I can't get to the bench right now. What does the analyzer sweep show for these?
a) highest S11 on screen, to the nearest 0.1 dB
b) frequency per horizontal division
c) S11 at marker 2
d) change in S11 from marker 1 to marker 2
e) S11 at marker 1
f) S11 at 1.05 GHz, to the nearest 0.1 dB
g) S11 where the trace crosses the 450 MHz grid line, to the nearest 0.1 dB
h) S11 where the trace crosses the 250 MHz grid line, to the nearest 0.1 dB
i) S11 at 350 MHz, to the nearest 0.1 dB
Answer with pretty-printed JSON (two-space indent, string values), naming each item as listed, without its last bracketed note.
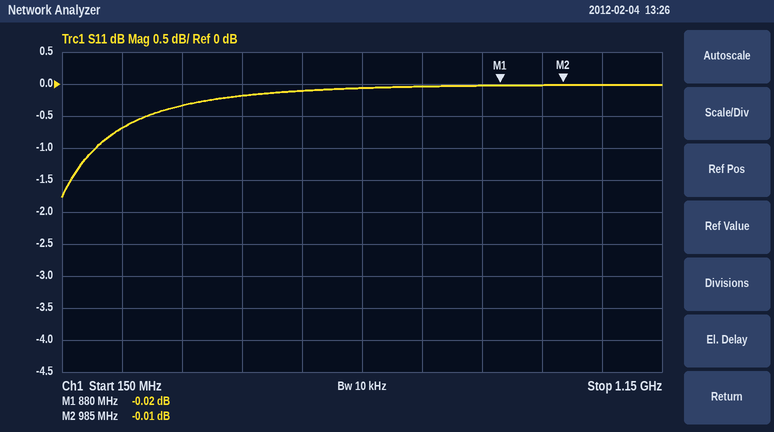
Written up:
{
  "highest S11 on screen, to the nearest 0.1 dB": "0.0 dB",
  "frequency per horizontal division": "100 MHz",
  "S11 at marker 2": "-0.01 dB",
  "change in S11 from marker 1 to marker 2": "0.01 dB",
  "S11 at marker 1": "-0.02 dB",
  "S11 at 1.05 GHz, to the nearest 0.1 dB": "0.0 dB",
  "S11 where the trace crosses the 450 MHz grid line, to the nearest 0.1 dB": "-0.2 dB",
  "S11 where the trace crosses the 250 MHz grid line, to the nearest 0.1 dB": "-0.7 dB",
  "S11 at 350 MHz, to the nearest 0.1 dB": "-0.3 dB"
}
